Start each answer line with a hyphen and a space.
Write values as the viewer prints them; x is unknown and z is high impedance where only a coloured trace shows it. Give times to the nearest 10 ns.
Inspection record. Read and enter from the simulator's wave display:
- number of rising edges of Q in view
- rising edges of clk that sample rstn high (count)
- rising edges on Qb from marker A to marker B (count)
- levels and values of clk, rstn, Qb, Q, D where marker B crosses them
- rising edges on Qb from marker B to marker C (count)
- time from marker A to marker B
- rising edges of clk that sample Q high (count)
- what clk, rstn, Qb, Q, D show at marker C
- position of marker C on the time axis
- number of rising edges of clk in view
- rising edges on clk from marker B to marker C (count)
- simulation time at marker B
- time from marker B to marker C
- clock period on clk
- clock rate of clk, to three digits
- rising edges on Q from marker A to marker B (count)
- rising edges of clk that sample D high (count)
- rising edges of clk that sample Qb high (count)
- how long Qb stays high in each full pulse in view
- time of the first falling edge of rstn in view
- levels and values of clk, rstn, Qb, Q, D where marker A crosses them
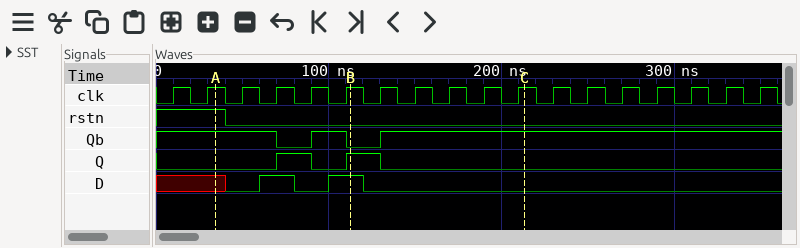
- 2
- 2
- 1
- clk=1, rstn=0, Qb=0, Q=1, D=1
- 1
- 80 ns
- 2
- clk=1, rstn=0, Qb=1, Q=0, D=0
- 210 ns
- 18
- 5
- 110 ns
- 100 ns
- 20 ns
- 50.0 MHz
- 2
- 2
- 16
- 20 ns
- 40 ns
- clk=1, rstn=1, Qb=1, Q=0, D=x
